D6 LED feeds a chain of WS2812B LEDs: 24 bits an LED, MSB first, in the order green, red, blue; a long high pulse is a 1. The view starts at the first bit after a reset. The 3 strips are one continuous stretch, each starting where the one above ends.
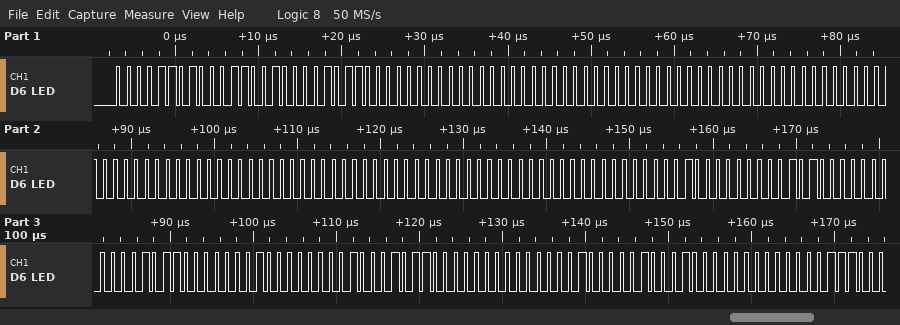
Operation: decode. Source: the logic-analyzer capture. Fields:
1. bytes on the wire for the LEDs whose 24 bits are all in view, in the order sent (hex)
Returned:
0D 19 0B 00 00 00 00 00 00 00 00 00 00 00 00 00 10 05 00 16 02 01 16 00 04 11 00
